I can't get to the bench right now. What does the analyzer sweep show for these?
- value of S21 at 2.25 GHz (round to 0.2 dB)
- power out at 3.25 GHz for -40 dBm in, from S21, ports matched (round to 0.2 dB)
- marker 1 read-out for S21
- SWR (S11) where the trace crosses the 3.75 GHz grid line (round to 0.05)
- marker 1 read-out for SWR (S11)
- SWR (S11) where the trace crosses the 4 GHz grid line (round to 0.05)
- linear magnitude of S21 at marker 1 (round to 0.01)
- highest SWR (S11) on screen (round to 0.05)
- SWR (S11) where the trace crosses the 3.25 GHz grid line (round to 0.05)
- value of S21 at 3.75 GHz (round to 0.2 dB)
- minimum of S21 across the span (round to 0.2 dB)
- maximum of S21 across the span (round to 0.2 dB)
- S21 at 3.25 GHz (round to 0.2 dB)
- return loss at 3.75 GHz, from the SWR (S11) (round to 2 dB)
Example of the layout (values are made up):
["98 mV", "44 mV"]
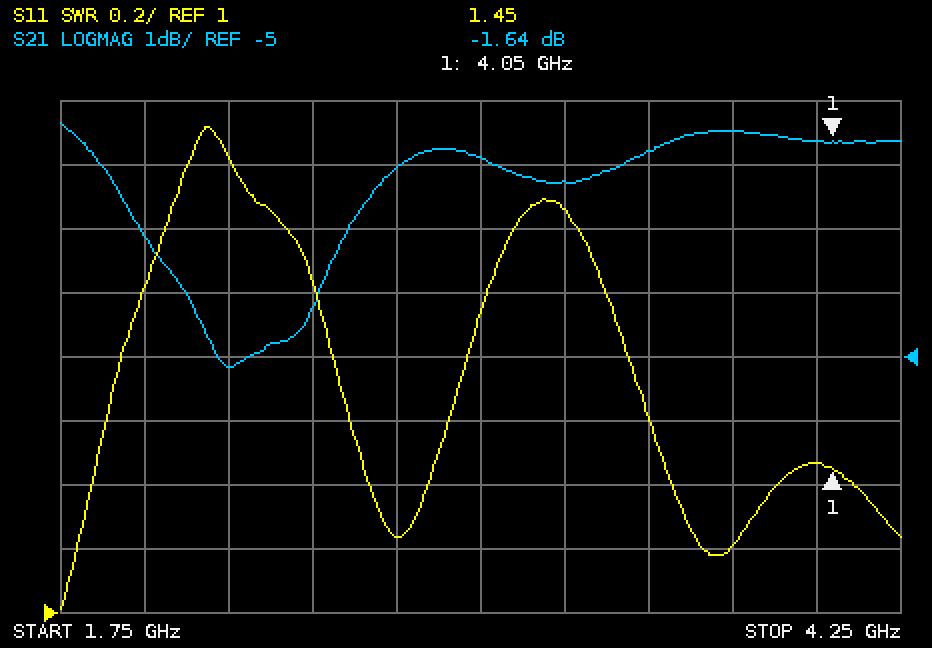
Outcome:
["-5.2 dB", "-42.2 dBm", "-1.64 dB", "1.20", "1.45", "1.45", "0.83", "2.50", "2.25", "-1.4 dB", "-5.2 dB", "-1.4 dB", "-2.2 dB", "20 dB"]
